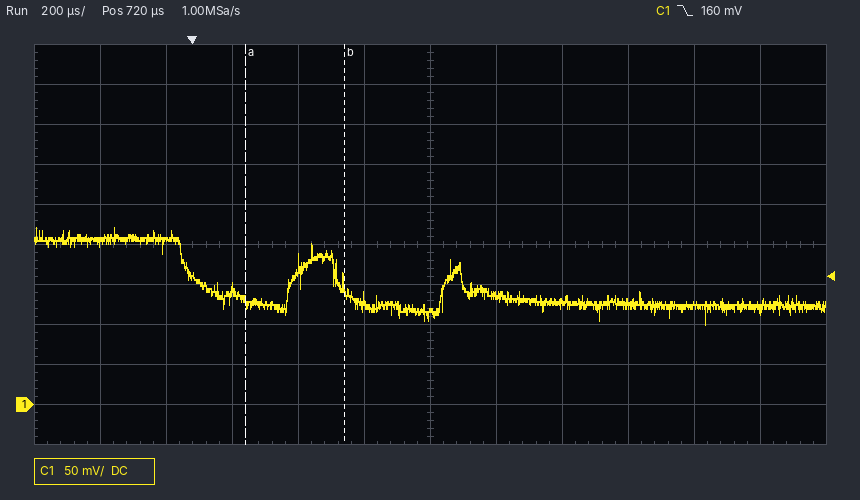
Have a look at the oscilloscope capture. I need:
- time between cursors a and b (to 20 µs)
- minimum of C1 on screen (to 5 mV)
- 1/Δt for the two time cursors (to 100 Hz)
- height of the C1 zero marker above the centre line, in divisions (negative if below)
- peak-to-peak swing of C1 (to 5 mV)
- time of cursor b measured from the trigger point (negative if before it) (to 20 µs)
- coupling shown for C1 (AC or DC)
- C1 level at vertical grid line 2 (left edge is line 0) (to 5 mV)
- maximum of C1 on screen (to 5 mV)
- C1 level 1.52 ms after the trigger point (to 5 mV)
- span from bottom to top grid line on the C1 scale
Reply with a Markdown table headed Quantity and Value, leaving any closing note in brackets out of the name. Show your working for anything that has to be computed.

| Quantity | Value |
|---|---|
| time between cursors a and b | 300 µs |
| minimum of C1 on screen | 100 mV |
| 1/Δt for the two time cursors | 1 / 300 µs ≈ 3.3 kHz |
| height of the C1 zero marker above the centre line, in divisions | -4.0 div |
| peak-to-peak swing of C1 | 220 mV − (100 mV) = 120 mV |
| time of cursor b measured from the trigger point (negative if before it) | +460 µs |
| coupling shown for C1 | DC |
| C1 level at vertical grid line 2 (left edge is line 0) | 205 mV |
| maximum of C1 on screen | 220 mV |
| C1 level 1.52 ms after the trigger point | 125 mV |
| span from bottom to top grid line on the C1 scale | 500 mV |
